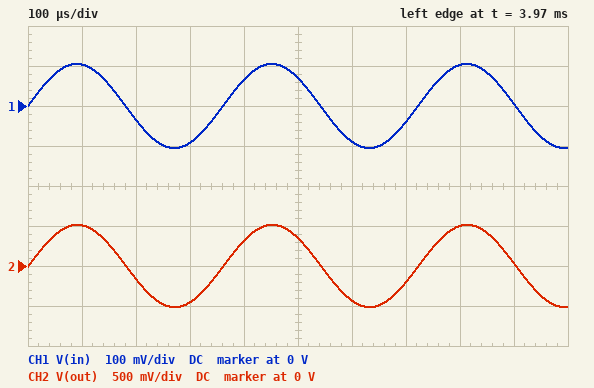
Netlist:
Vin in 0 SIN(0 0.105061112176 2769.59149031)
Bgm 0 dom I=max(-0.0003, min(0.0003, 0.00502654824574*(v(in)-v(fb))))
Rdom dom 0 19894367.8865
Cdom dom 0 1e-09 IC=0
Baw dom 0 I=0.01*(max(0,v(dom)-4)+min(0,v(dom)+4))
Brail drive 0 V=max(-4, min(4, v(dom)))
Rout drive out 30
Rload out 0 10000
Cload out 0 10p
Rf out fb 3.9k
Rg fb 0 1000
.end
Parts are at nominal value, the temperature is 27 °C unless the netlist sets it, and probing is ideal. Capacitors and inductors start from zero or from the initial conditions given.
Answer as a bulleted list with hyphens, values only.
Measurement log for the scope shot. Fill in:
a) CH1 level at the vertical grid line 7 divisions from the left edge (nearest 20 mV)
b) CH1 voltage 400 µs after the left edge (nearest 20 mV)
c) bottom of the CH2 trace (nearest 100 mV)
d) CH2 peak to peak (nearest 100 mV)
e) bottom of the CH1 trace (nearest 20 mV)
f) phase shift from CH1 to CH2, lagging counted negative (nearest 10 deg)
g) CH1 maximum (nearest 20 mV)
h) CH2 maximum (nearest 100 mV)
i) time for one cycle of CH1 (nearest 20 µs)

- -40 mV
- 60 mV
- -500 mV
- 1.0 V
- -100 mV
- 0 deg
- 100 mV
- 500 mV
- 360 µs
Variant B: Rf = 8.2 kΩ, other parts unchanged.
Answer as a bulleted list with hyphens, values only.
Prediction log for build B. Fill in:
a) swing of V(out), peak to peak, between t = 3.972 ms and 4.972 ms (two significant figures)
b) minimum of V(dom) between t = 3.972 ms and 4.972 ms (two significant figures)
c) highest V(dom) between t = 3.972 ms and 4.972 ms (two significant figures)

- 1.9 V
- -970 mV
- 970 mV
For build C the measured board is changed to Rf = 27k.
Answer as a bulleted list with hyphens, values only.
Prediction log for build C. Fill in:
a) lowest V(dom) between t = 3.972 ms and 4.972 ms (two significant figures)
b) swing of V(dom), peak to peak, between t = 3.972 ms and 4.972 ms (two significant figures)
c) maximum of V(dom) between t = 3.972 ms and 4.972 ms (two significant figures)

- -2.9 V
- 5.9 V
- 2.9 V
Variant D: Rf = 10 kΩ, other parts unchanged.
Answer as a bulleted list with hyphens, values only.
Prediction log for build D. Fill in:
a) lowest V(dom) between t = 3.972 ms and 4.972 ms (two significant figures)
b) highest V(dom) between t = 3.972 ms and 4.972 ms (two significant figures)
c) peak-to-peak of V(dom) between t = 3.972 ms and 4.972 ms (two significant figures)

- -1.2 V
- 1.2 V
- 2.3 V
